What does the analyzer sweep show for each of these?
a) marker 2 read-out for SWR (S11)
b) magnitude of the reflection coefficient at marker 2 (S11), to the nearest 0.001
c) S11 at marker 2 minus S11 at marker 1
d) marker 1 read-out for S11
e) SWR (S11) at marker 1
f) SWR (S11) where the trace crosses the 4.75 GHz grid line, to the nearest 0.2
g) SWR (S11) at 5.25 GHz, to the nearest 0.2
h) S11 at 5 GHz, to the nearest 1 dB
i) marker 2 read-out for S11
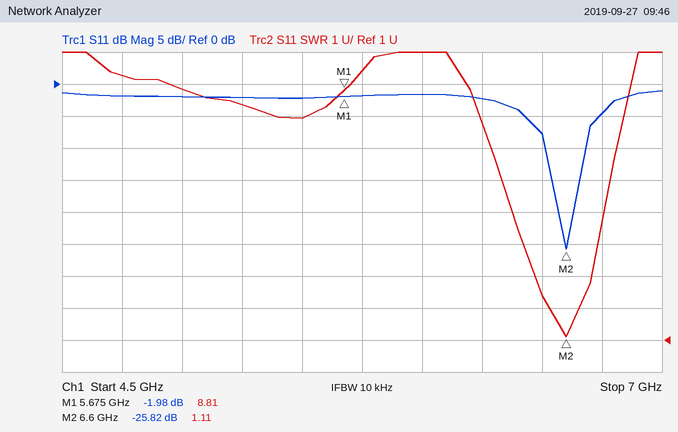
1.11
0.051
-23.84 dB
-1.98 dB
8.81
9.2
8.4
-2 dB
-25.82 dB
